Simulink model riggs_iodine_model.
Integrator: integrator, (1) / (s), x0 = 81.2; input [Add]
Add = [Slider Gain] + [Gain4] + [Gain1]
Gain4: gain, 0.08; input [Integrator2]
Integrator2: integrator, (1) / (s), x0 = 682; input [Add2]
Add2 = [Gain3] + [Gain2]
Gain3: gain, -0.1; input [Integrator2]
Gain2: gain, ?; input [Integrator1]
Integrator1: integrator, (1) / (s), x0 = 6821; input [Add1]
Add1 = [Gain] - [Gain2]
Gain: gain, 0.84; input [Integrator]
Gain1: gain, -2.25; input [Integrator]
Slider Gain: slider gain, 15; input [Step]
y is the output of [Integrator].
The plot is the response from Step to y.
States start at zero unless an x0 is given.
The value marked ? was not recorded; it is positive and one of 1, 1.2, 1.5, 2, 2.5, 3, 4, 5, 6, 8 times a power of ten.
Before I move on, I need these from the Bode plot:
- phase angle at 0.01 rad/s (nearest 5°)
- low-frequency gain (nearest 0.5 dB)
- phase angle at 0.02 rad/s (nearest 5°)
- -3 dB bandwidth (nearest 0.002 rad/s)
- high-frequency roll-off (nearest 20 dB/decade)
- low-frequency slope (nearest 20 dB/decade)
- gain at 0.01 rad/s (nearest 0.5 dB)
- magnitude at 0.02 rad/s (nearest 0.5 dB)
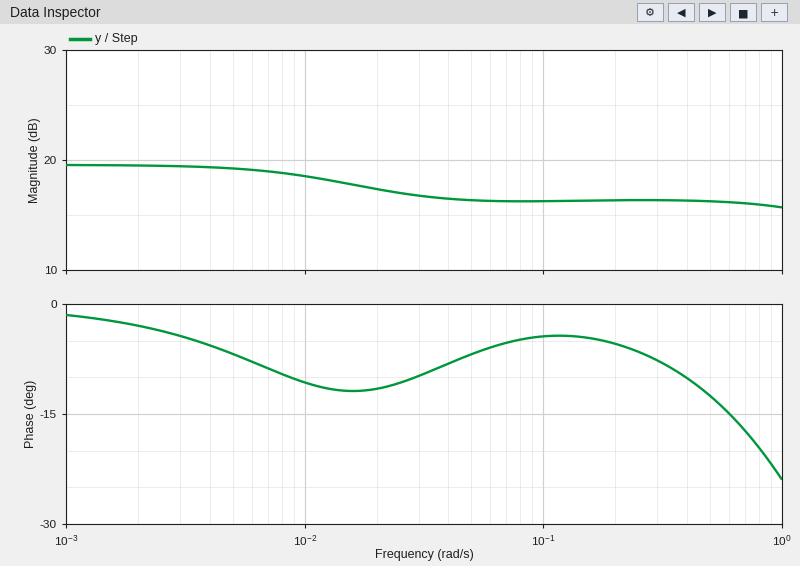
-10°
19.5 dB
-10°
0.038 rad/s
0 dB/decade
0 dB/decade
18.5 dB
17.5 dB
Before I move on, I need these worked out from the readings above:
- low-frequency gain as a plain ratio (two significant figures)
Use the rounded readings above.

9.4
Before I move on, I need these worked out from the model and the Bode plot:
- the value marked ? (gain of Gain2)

0.02
